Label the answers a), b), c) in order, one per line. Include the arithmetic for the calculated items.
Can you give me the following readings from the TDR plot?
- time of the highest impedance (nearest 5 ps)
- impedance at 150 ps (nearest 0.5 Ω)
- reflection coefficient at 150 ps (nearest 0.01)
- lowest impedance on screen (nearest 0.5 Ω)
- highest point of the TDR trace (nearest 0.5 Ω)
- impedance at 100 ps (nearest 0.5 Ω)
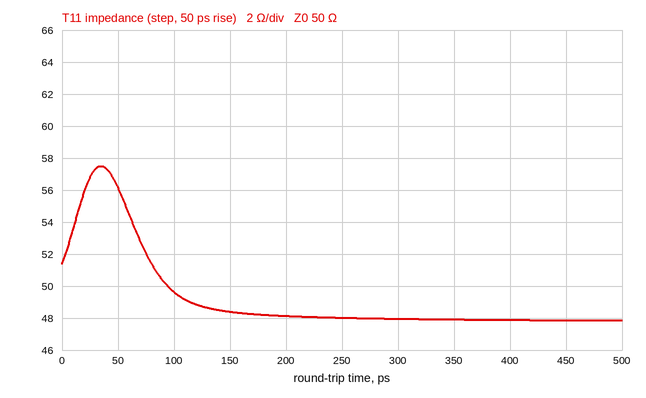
a) 35 ps
b) 48.5 Ω
c) (48.5 − 50)/(48.5 + 50) ≈ -0.02
d) 48.0 Ω
e) 57.5 Ω
f) 49.5 Ω
